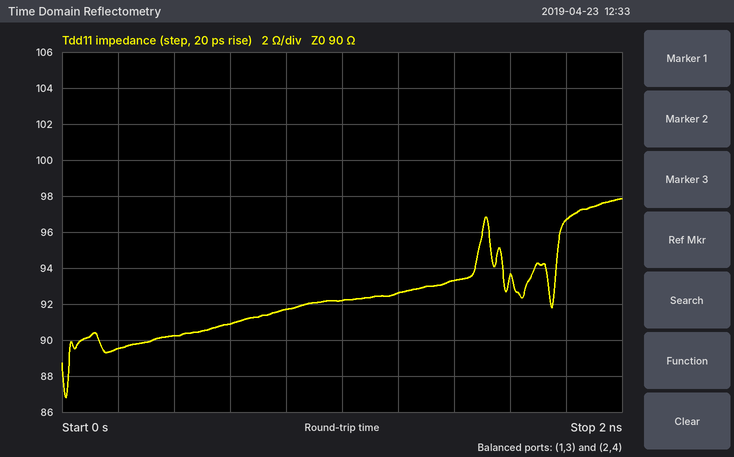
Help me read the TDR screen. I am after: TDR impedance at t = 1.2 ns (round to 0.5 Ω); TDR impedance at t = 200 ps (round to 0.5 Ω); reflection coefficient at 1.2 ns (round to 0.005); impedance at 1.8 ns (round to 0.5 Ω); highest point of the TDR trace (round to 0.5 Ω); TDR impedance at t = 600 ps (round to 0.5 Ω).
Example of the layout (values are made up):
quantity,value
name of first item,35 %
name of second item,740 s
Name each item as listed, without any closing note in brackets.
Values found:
quantity,value
TDR impedance at t = 1.2 ns,92.5 Ω
TDR impedance at t = 200 ps,89.5 Ω
reflection coefficient at 1.2 ns,+0.015
impedance at 1.8 ns,96.5 Ω
highest point of the TDR trace,98.0 Ω
TDR impedance at t = 600 ps,91.0 Ω
